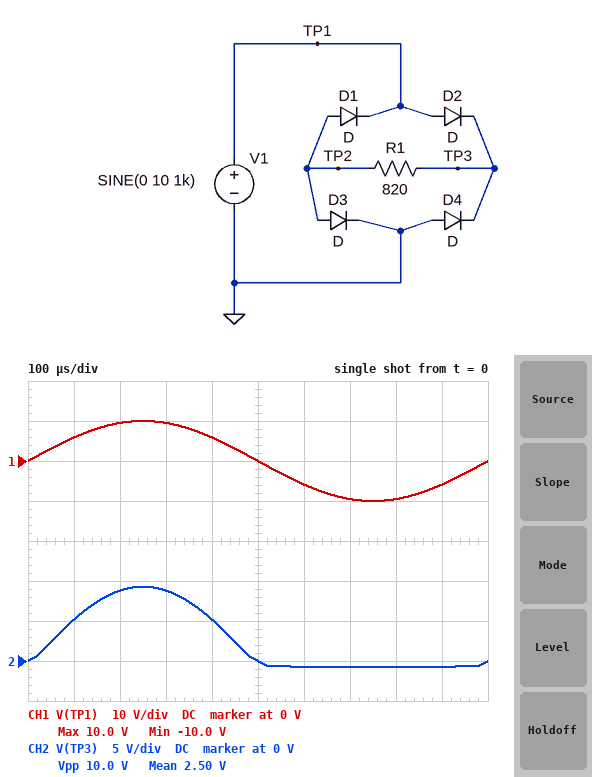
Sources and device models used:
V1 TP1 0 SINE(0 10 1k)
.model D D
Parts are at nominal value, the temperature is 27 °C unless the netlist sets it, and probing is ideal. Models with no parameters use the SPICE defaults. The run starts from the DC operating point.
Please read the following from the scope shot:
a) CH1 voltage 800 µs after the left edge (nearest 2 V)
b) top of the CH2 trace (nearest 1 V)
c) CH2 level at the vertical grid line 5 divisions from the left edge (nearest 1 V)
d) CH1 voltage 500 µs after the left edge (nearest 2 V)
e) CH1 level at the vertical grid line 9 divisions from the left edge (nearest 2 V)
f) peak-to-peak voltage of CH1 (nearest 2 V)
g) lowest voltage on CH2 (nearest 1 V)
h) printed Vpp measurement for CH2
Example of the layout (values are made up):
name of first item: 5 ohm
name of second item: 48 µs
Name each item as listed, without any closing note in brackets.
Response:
CH1 voltage 800 µs after the left edge: -10 V
top of the CH2 trace: 9 V
CH2 level at the vertical grid line 5 divisions from the left edge: 0 V
CH1 voltage 500 µs after the left edge: 0 V
CH1 level at the vertical grid line 9 divisions from the left edge: -6 V
peak-to-peak voltage of CH1: 20 V
lowest voltage on CH2: -1 V
printed Vpp measurement for CH2: 10.0 V
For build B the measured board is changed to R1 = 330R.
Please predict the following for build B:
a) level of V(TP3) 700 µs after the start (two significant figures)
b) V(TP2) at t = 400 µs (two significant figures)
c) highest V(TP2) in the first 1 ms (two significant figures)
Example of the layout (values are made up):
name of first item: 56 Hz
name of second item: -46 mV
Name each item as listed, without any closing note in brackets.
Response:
level of V(TP3) 700 µs after the start: -740 mV
V(TP2) at t = 400 µs: 720 mV
highest V(TP2) in the first 1 ms: 740 mV
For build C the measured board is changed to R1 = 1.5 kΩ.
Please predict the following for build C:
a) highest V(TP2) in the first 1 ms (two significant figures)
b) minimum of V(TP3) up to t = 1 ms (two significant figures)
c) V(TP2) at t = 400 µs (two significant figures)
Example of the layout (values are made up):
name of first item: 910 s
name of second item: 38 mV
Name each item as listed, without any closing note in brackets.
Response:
highest V(TP2) in the first 1 ms: 700 mV
minimum of V(TP3) up to t = 1 ms: -700 mV
V(TP2) at t = 400 µs: 680 mV
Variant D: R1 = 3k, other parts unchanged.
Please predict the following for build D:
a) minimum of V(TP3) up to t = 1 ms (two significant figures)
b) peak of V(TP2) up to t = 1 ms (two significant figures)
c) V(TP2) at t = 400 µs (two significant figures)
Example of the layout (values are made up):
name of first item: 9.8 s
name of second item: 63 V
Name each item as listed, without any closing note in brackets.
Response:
minimum of V(TP3) up to t = 1 ms: -680 mV
peak of V(TP2) up to t = 1 ms: 680 mV
V(TP2) at t = 400 µs: 670 mV
